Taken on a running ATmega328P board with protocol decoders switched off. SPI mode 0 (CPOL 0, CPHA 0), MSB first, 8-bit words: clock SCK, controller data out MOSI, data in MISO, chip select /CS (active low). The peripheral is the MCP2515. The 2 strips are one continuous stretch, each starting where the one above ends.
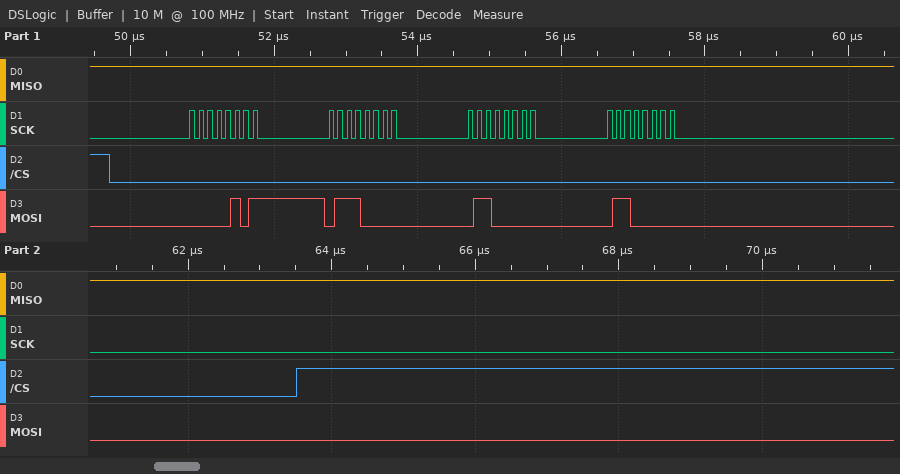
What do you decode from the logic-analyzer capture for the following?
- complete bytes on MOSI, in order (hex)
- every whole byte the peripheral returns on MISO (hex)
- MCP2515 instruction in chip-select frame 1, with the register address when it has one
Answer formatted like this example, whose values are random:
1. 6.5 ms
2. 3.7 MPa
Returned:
1. 05 70 60 60
2. FF FF FF FF
3. BIT MODIFY 0x70
